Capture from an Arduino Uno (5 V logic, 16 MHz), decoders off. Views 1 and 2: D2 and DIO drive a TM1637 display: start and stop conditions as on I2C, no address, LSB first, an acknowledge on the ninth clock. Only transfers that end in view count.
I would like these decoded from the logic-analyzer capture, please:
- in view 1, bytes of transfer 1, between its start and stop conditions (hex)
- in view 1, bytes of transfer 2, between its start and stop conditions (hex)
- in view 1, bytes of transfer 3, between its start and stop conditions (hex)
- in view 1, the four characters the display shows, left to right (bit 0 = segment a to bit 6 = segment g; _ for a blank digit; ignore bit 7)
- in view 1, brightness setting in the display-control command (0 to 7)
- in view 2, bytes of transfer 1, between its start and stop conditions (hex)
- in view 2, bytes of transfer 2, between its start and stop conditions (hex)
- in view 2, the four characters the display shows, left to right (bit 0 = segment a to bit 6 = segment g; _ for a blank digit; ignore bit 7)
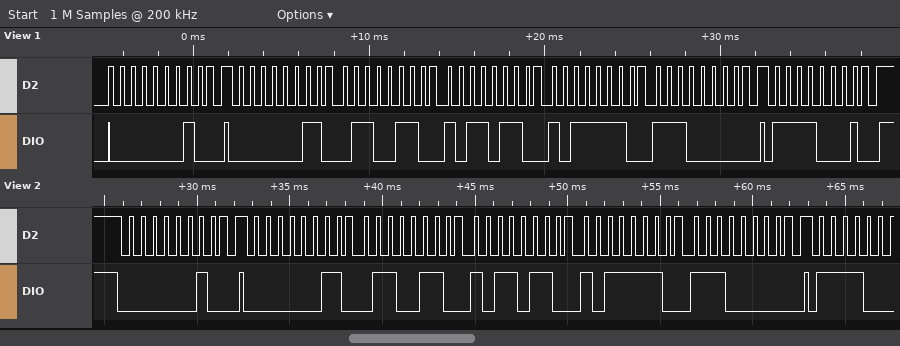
40
C0 66 6D 7D 07
8F
4567
7
40
C0 66 6D 7D 07
4567
